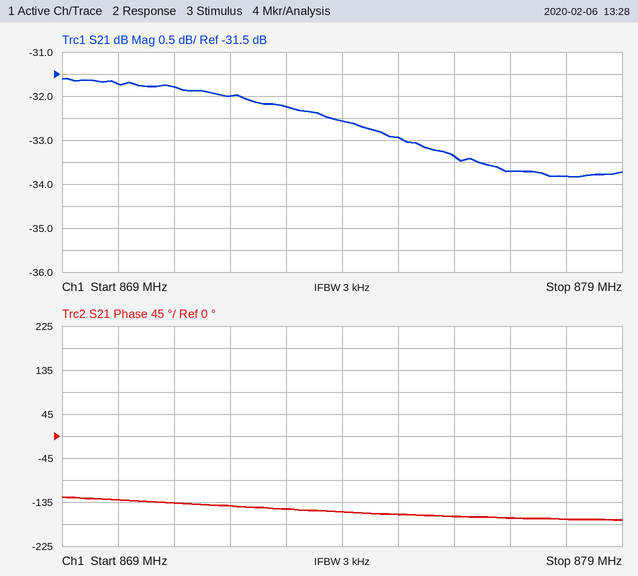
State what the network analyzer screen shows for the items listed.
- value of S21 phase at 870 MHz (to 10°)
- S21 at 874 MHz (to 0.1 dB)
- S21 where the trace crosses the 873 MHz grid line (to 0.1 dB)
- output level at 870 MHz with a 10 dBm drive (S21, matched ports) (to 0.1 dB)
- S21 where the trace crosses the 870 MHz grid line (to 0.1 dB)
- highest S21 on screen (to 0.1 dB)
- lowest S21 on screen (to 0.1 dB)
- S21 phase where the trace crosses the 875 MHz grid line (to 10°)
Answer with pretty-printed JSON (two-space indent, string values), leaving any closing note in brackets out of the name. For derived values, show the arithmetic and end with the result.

{
  "value of S21 phase at 870 MHz": "-130°",
  "S21 at 874 MHz": "-32.6 dB",
  "S21 where the trace crosses the 873 MHz grid line": "-32.2 dB",
  "output level at 870 MHz with a 10 dBm drive (S21, matched ports)": "10 dBm + (-31.7 dB) = -21.7 dBm",
  "S21 where the trace crosses the 870 MHz grid line": "-31.7 dB",
  "highest S21 on screen": "-31.6 dB",
  "lowest S21 on screen": "-33.8 dB",
  "S21 phase where the trace crosses the 875 MHz grid line": "-160°"
}
